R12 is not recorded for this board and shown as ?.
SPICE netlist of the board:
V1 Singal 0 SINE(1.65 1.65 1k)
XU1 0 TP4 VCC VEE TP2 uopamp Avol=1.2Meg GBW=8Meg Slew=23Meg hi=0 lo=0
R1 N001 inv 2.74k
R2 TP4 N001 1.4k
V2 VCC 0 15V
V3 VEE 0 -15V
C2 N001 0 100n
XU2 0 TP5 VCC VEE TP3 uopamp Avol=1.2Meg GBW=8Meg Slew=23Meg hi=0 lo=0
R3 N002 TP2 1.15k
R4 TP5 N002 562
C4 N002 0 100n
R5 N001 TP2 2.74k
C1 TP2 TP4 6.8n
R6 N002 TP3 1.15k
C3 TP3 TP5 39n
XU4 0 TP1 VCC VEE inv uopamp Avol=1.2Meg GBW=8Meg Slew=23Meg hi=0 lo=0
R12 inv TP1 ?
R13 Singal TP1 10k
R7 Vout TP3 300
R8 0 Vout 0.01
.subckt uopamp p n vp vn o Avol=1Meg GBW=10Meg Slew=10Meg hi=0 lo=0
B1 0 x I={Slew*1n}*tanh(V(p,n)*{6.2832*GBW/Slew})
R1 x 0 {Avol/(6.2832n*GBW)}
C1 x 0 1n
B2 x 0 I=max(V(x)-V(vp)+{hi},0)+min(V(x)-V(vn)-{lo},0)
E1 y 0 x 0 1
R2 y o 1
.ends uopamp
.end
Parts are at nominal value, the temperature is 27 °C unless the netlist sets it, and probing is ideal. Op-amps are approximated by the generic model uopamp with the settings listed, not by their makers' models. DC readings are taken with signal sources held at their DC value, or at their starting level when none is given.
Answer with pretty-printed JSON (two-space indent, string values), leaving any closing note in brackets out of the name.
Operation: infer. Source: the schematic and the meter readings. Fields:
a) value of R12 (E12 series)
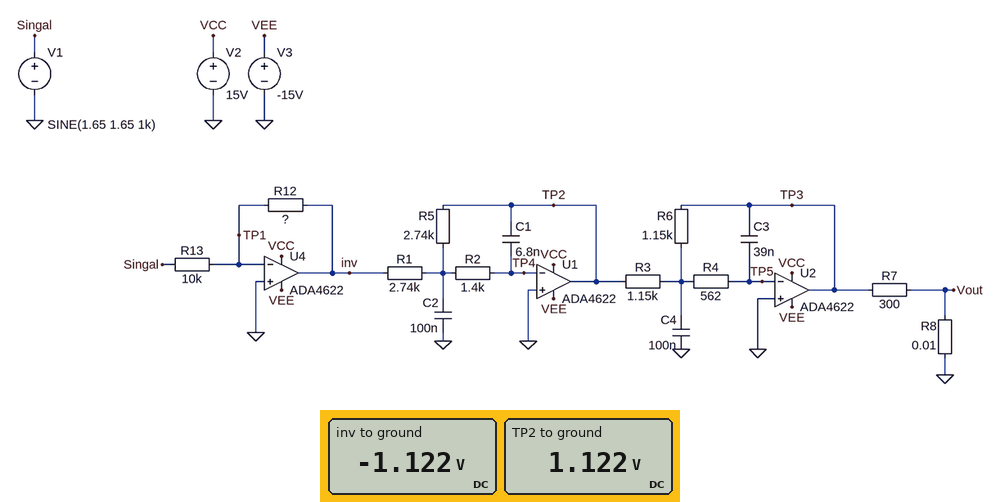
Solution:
{
  "value of R12": "6.8 kΩ"
}
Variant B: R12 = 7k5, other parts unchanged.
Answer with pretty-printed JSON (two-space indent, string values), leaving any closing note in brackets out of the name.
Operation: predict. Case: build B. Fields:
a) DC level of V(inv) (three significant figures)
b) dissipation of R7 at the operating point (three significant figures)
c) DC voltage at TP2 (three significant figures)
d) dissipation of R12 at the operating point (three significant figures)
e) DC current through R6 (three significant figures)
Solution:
{
  "DC level of V(inv)": "-1.24 V",
  "dissipation of R7 at the operating point": "5.10 mW",
  "DC voltage at TP2": "1.24 V",
  "dissipation of R12 at the operating point": "204 µW",
  "DC current through R6": "1.08 mA"
}
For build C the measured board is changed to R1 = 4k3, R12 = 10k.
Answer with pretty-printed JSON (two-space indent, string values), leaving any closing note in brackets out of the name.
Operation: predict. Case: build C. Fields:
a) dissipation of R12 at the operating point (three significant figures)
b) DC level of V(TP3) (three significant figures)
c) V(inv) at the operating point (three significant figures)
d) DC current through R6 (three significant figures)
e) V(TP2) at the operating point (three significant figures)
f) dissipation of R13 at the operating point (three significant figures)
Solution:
{
  "dissipation of R12 at the operating point": "272 µW",
  "DC level of V(TP3)": "-1.05 V",
  "V(inv) at the operating point": "-1.65 V",
  "DC current through R6": "914 µA",
  "V(TP2) at the operating point": "1.05 V",
  "dissipation of R13 at the operating point": "272 µW"
}
